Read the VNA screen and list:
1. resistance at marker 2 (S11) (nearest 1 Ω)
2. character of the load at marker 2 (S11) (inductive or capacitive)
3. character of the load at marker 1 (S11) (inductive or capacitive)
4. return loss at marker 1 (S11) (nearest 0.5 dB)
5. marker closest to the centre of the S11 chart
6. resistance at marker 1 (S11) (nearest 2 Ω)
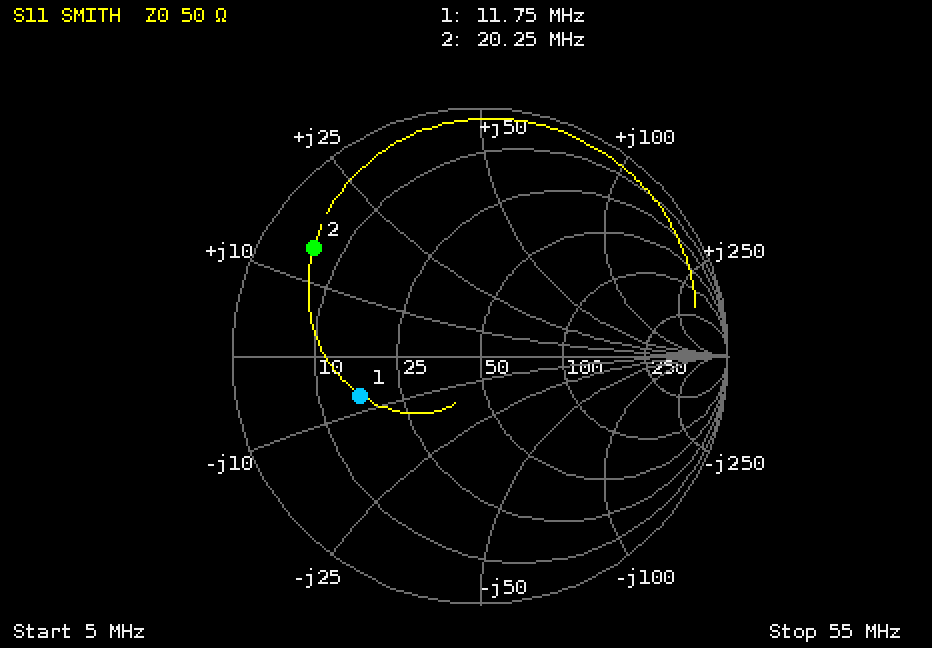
6 Ω
inductive
capacitive
6.0 dB
marker 1
16 Ω
